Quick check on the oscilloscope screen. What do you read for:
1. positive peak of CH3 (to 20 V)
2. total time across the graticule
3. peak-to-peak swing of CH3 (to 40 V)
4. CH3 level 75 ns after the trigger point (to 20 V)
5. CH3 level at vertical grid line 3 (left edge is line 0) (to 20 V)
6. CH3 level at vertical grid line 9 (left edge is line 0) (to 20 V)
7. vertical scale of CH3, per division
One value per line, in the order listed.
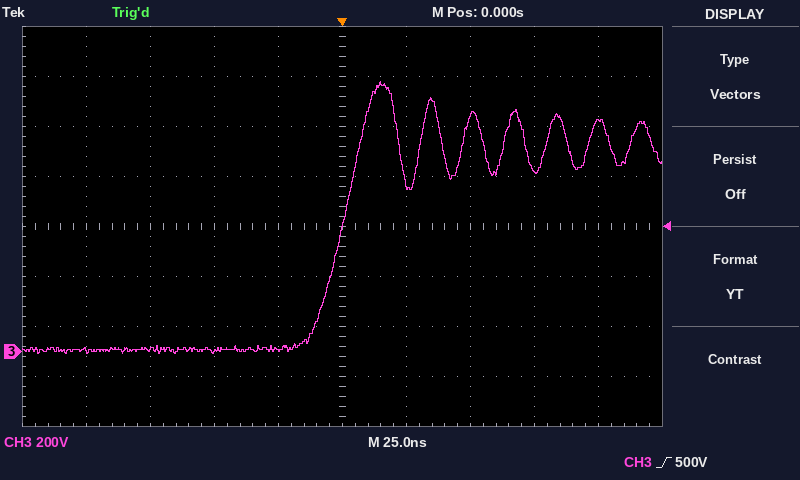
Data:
1.08 kV
250 ns
1.08 kV
720 V
0 V
920 V
200 V
